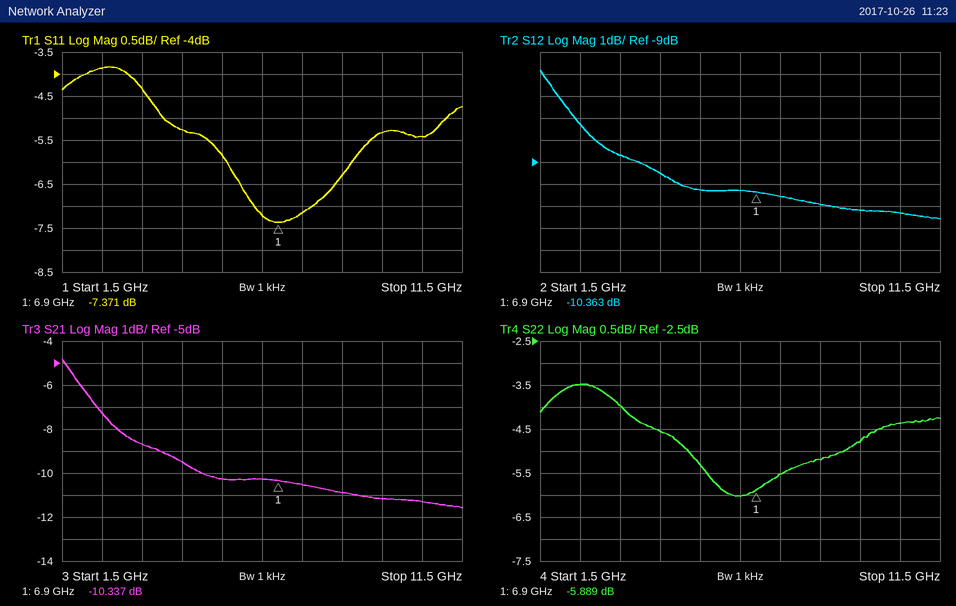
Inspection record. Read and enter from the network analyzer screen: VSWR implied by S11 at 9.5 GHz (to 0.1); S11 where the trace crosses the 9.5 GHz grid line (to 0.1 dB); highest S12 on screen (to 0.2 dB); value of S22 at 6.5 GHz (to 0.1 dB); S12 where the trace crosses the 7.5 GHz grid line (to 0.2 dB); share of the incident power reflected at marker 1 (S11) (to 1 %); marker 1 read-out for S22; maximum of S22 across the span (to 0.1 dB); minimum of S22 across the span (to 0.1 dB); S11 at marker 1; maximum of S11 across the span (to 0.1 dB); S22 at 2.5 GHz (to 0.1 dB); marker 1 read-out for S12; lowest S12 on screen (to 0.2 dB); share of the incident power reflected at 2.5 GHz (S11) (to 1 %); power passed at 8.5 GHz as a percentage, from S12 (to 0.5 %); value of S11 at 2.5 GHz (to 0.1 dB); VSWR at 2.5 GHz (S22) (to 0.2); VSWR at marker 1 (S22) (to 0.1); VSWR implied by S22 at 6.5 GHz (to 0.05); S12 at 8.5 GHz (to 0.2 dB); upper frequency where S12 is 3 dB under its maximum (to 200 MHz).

3.4
-5.3 dB
-4.8 dB
-6.0 dB
-10.6 dB
18 %
-5.889 dB
-3.5 dB
-6.0 dB
-7.371 dB
-3.8 dB
-3.5 dB
-10.363 dB
-11.6 dB
41 %
8.0 %
-3.9 dB
5.0
3.1
3.00
-11.0 dB
2.8 GHz
